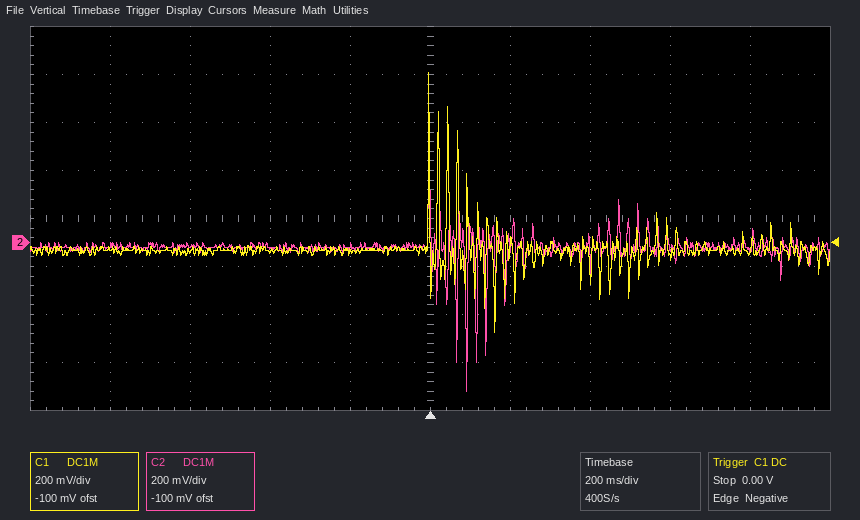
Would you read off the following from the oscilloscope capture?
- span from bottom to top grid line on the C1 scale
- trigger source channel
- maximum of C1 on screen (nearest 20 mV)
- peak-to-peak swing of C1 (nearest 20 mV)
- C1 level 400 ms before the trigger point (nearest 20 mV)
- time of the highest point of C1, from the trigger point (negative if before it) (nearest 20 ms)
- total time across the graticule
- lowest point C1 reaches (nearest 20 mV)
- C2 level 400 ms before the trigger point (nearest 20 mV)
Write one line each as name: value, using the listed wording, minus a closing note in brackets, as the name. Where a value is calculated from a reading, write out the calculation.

span from bottom to top grid line on the C1 scale: 1.6 V
trigger source channel: C1
maximum of C1 on screen: 700 mV
peak-to-peak swing of C1: 700 mV − (-380 mV) = 1.08 V
C1 level 400 ms before the trigger point: -40 mV
time of the highest point of C1, from the trigger point (negative if before it): 0 ms
total time across the graticule: 2 s
lowest point C1 reaches: -380 mV
C2 level 400 ms before the trigger point: -20 mV
